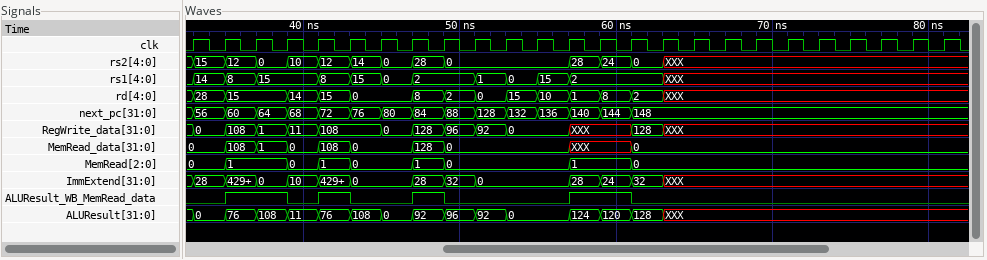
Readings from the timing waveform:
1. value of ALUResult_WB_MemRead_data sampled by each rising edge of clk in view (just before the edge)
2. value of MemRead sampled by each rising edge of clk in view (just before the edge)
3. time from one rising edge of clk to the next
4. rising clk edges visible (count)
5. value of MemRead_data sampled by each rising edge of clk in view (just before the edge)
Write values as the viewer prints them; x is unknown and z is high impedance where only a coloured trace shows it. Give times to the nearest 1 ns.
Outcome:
0 0 1 1 0 1 0 0 1 0 0 0 0 1 1 0 0 0 0 0 0 0 0 0 0
0, 0, 1, 1, 0, 1, 0, 0, 1, 0, 0, 0, 0, 1, 1, 0, 0, 0, 0, 0, 0, 0, 0, 0, 0
2 ns
25
0, 0, 108, 1, 0, 108, 0, 0, 128, 0, 0, 0, 0, XXX, XXX, 0, 0, 0, 0, 0, 0, 0, 0, 0, 0
